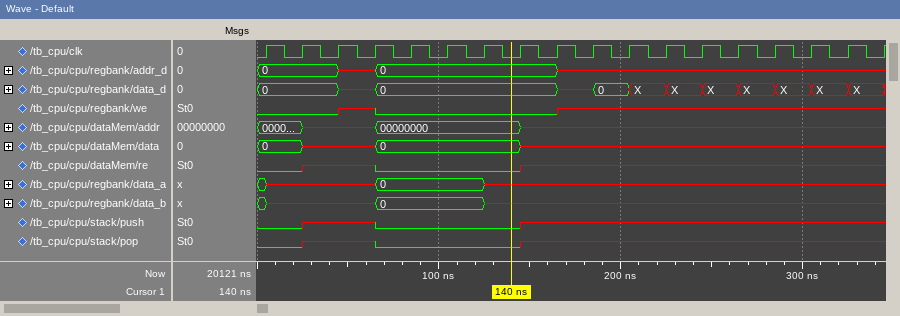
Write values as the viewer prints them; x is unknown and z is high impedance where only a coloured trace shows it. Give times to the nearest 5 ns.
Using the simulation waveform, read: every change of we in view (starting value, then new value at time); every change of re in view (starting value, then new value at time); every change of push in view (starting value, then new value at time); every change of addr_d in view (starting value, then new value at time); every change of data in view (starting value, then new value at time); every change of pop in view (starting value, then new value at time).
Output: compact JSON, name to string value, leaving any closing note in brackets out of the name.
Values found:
{"every change of we in view": "0, x at 45 ns, 0 at 65 ns, x at 165 ns", "every change of re in view": "0, x at 25 ns, 0 at 65 ns, x at 145 ns", "every change of push in view": "0, x at 25 ns, 0 at 65 ns, x at 145 ns", "every change of addr_d in view": "0, x at 45 ns, 0 at 65 ns, x at 165 ns", "every change of data in view": "0, x at 25 ns, 0 at 65 ns, x at 145 ns", "every change of pop in view": "0, x at 25 ns, 0 at 65 ns, x at 145 ns"}
